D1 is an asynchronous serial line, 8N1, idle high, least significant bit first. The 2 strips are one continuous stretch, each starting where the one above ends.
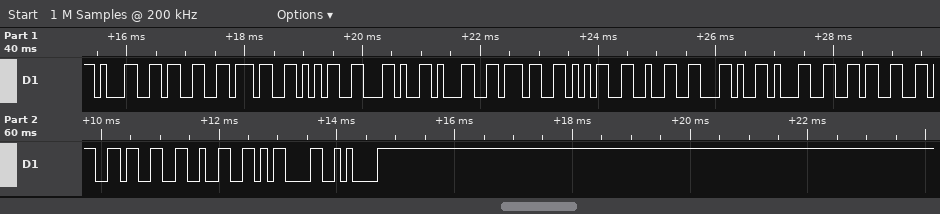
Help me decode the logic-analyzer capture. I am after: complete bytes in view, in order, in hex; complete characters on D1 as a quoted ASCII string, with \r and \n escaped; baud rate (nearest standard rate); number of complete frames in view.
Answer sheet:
31 33 37 35 2C 31 37 35 32 2C 31 36 36 33 32 0D 0A
"1375,1752,16632\r\n"
9600 baud
17
